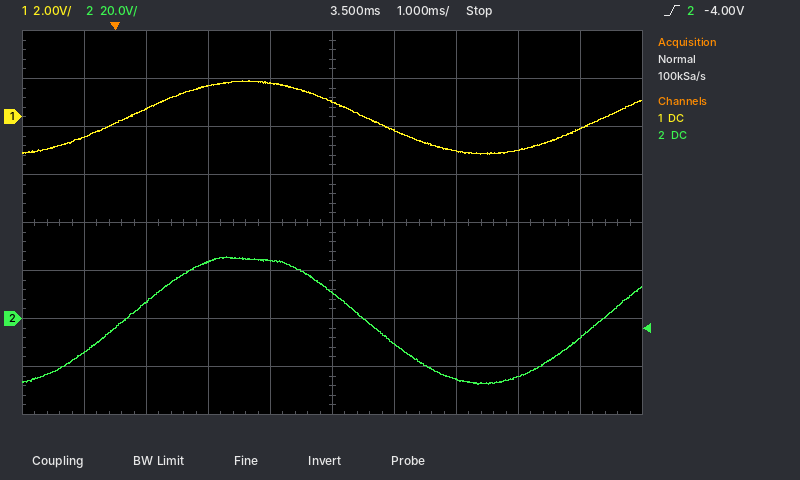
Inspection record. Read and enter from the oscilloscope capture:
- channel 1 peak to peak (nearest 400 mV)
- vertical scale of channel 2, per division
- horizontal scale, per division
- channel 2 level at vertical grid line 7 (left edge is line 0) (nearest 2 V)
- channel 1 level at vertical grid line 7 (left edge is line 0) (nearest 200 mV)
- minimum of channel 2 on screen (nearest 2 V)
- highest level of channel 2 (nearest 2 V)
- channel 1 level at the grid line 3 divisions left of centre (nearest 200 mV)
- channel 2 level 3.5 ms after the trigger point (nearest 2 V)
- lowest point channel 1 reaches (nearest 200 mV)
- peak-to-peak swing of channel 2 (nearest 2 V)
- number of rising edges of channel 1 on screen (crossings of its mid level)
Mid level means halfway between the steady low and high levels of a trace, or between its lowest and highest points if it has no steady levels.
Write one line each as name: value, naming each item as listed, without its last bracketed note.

channel 1 peak to peak: 3.2 V
vertical scale of channel 2, per division: 20 V
horizontal scale, per division: 1 ms
channel 2 level at vertical grid line 7 (left edge is line 0): -26 V
channel 1 level at vertical grid line 7 (left edge is line 0): -1.4 V
minimum of channel 2 on screen: -28 V
highest level of channel 2: 26 V
channel 1 level at the grid line 3 divisions left of centre: 400 mV
channel 2 level 3.5 ms after the trigger point: 10 V
lowest point channel 1 reaches: -1.6 V
peak-to-peak swing of channel 2: 54 V
number of rising edges of channel 1 on screen: 2
